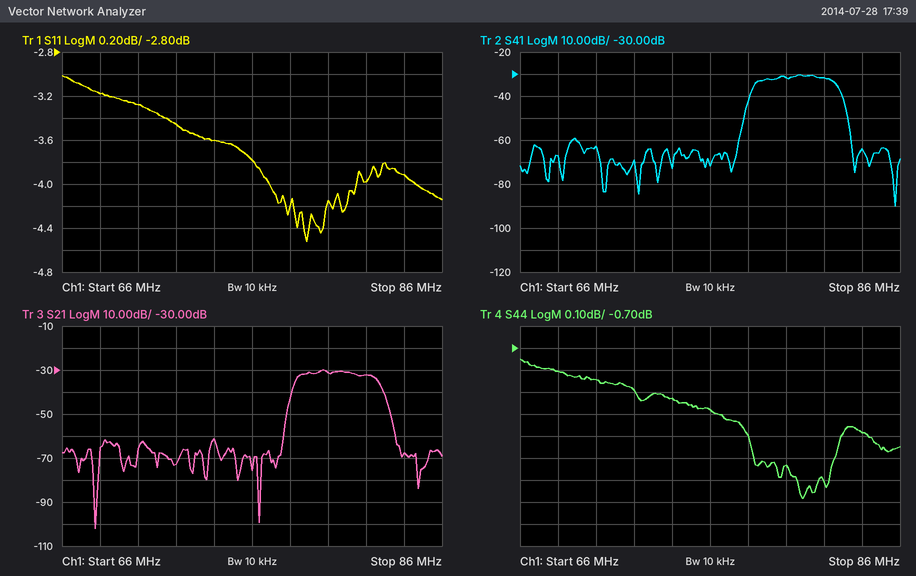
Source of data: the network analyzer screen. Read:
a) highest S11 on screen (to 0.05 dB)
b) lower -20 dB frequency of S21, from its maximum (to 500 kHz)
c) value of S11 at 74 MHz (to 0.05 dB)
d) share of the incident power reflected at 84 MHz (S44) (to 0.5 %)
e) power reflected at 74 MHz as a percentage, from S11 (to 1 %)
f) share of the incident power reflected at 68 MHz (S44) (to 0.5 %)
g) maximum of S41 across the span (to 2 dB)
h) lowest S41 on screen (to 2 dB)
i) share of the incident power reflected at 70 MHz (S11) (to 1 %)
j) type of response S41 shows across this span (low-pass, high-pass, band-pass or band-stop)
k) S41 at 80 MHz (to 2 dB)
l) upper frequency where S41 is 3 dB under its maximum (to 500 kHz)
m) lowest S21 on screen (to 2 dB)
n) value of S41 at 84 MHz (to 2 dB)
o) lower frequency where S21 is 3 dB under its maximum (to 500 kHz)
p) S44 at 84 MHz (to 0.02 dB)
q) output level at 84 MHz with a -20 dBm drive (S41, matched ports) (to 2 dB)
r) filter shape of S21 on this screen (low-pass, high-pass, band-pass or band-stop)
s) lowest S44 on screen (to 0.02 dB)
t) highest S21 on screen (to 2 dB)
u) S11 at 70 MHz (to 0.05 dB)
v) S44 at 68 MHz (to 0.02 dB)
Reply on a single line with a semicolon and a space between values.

-3.00 dB; 78.0 MHz; -3.60 dB; 78.0 %; 44 %; 83.0 %; -30 dB; -90 dB; 47 %; band-pass; -32 dB; 82.5 MHz; -102 dB; -64 dB; 78.5 MHz; -1.08 dB; -84 dBm; band-pass; -1.38 dB; -30 dB; -3.30 dB; -0.80 dB
